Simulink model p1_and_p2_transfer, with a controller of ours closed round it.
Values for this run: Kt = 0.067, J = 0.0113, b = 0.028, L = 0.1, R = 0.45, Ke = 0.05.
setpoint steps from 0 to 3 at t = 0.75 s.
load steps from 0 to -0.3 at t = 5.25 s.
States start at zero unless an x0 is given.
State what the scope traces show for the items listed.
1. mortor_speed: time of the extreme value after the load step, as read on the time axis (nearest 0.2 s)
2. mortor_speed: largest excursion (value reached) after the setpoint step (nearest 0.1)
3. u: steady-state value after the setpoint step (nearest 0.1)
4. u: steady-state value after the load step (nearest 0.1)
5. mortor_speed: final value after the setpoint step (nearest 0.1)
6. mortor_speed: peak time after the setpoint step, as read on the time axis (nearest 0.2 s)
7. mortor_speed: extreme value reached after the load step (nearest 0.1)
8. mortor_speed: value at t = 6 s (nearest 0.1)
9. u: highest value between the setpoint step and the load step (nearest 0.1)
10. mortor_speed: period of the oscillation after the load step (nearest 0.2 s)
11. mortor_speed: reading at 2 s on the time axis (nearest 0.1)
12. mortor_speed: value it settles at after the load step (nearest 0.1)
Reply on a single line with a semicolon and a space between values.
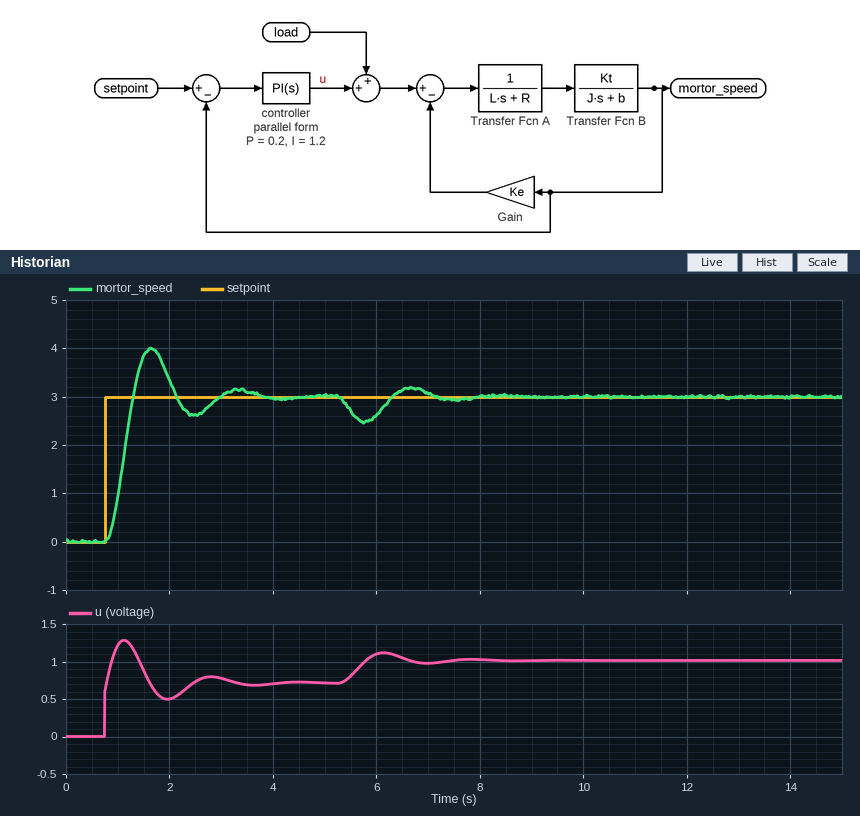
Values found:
5.8 s; 4.0; 0.7; 1.0; 3.0; 1.6 s; 2.5; 2.6; 1.3; 1.8 s; 3.3; 3.0
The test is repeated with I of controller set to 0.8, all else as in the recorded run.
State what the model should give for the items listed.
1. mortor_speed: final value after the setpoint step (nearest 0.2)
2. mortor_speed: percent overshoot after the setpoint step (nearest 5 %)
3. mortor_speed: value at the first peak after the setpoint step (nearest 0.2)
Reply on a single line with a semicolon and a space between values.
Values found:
3.0; 15 %; 3.4
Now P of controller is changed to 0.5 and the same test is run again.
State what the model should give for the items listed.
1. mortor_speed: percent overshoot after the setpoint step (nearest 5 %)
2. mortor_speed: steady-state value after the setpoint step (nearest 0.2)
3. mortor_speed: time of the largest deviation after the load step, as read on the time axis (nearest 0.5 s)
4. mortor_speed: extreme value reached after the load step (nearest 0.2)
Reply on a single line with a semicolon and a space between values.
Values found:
15 %; 3.0; 5.5 s; 2.6
